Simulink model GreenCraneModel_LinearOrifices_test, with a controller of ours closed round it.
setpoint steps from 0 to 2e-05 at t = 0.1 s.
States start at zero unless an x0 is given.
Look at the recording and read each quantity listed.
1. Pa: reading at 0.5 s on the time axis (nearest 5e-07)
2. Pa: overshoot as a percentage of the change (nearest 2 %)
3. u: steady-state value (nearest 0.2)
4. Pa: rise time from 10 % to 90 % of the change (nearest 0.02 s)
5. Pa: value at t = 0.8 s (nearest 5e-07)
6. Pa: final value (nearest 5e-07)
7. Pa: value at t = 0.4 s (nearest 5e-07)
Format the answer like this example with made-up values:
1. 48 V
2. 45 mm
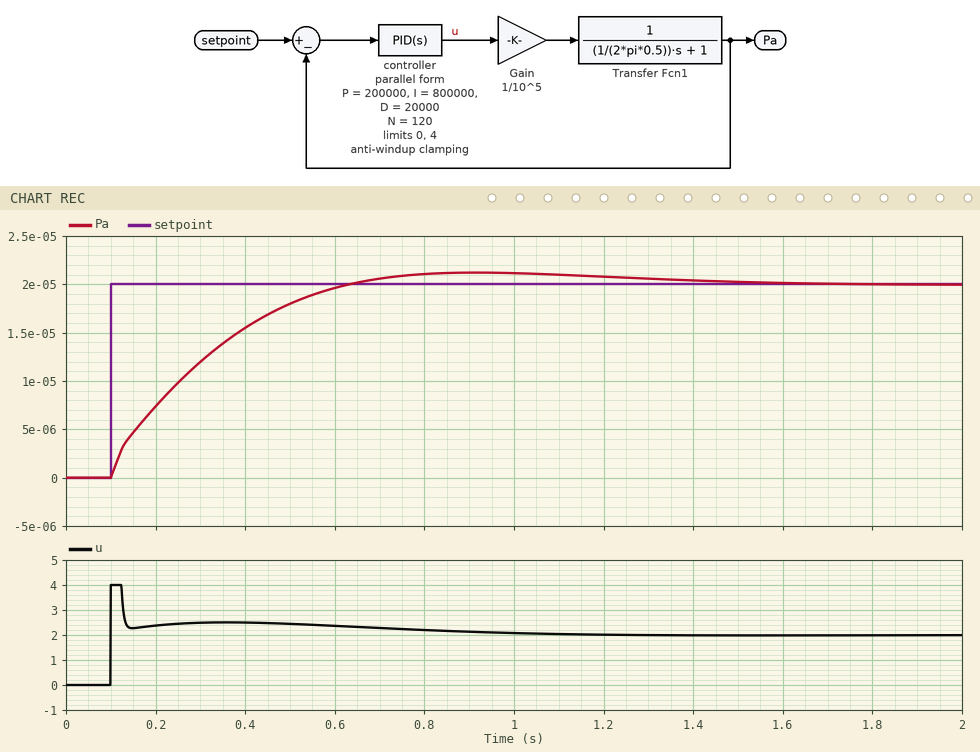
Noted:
1. 0.0000180
2. 6 %
3. 2.0
4. 0.38 s
5. 0.0000210
6. 0.0000200
7. 0.0000155
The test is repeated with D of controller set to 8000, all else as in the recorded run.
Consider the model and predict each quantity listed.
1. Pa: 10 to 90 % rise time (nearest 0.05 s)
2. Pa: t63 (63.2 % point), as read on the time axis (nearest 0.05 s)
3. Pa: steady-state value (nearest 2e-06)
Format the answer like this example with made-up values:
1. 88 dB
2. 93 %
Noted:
1. 0.35 s
2. 0.30 s
3. 0.000020
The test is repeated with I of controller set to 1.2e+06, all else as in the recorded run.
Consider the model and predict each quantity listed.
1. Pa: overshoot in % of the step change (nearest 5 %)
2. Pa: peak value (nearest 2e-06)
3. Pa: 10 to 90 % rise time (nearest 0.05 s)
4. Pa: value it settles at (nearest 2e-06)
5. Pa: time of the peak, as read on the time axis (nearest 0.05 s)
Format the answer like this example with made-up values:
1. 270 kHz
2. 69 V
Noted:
1. 10 %
2. 0.000022
3. 0.30 s
4. 0.000020
5. 0.75 s
